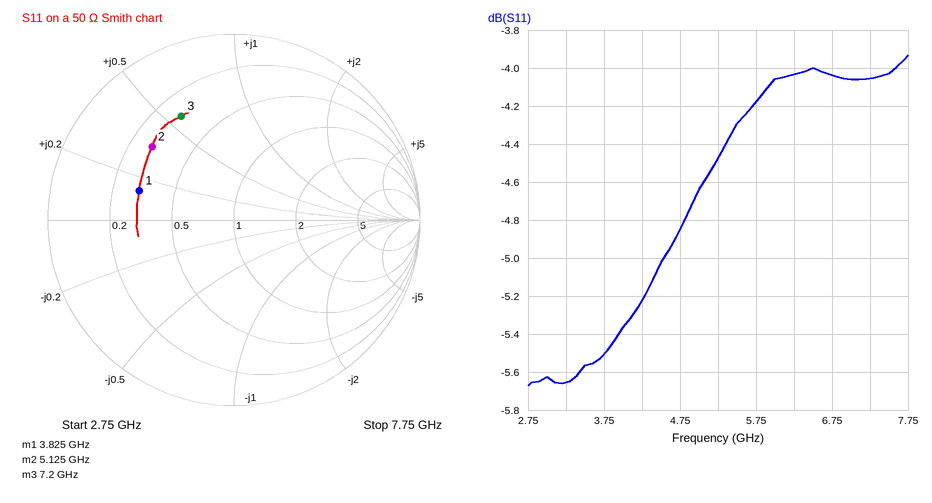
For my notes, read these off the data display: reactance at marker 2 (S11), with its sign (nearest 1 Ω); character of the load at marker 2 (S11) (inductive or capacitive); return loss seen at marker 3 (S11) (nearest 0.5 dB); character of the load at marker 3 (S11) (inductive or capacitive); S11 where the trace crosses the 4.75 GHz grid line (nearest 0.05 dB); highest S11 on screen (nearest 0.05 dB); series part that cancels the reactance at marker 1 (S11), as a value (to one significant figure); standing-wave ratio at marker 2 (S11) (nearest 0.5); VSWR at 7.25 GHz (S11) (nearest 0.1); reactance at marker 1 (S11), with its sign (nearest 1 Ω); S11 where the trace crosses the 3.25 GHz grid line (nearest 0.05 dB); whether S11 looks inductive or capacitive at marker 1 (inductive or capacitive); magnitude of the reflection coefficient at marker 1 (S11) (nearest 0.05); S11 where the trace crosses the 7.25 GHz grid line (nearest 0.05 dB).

+18 Ω
inductive
4.0 dB
inductive
-4.85 dB
-3.95 dB
6 pF
4.0
4.4
+7 Ω
-5.65 dB
inductive
0.55
-4.05 dB
